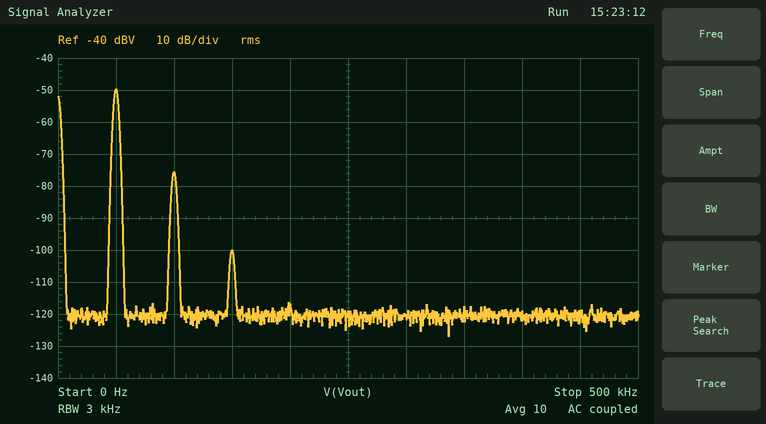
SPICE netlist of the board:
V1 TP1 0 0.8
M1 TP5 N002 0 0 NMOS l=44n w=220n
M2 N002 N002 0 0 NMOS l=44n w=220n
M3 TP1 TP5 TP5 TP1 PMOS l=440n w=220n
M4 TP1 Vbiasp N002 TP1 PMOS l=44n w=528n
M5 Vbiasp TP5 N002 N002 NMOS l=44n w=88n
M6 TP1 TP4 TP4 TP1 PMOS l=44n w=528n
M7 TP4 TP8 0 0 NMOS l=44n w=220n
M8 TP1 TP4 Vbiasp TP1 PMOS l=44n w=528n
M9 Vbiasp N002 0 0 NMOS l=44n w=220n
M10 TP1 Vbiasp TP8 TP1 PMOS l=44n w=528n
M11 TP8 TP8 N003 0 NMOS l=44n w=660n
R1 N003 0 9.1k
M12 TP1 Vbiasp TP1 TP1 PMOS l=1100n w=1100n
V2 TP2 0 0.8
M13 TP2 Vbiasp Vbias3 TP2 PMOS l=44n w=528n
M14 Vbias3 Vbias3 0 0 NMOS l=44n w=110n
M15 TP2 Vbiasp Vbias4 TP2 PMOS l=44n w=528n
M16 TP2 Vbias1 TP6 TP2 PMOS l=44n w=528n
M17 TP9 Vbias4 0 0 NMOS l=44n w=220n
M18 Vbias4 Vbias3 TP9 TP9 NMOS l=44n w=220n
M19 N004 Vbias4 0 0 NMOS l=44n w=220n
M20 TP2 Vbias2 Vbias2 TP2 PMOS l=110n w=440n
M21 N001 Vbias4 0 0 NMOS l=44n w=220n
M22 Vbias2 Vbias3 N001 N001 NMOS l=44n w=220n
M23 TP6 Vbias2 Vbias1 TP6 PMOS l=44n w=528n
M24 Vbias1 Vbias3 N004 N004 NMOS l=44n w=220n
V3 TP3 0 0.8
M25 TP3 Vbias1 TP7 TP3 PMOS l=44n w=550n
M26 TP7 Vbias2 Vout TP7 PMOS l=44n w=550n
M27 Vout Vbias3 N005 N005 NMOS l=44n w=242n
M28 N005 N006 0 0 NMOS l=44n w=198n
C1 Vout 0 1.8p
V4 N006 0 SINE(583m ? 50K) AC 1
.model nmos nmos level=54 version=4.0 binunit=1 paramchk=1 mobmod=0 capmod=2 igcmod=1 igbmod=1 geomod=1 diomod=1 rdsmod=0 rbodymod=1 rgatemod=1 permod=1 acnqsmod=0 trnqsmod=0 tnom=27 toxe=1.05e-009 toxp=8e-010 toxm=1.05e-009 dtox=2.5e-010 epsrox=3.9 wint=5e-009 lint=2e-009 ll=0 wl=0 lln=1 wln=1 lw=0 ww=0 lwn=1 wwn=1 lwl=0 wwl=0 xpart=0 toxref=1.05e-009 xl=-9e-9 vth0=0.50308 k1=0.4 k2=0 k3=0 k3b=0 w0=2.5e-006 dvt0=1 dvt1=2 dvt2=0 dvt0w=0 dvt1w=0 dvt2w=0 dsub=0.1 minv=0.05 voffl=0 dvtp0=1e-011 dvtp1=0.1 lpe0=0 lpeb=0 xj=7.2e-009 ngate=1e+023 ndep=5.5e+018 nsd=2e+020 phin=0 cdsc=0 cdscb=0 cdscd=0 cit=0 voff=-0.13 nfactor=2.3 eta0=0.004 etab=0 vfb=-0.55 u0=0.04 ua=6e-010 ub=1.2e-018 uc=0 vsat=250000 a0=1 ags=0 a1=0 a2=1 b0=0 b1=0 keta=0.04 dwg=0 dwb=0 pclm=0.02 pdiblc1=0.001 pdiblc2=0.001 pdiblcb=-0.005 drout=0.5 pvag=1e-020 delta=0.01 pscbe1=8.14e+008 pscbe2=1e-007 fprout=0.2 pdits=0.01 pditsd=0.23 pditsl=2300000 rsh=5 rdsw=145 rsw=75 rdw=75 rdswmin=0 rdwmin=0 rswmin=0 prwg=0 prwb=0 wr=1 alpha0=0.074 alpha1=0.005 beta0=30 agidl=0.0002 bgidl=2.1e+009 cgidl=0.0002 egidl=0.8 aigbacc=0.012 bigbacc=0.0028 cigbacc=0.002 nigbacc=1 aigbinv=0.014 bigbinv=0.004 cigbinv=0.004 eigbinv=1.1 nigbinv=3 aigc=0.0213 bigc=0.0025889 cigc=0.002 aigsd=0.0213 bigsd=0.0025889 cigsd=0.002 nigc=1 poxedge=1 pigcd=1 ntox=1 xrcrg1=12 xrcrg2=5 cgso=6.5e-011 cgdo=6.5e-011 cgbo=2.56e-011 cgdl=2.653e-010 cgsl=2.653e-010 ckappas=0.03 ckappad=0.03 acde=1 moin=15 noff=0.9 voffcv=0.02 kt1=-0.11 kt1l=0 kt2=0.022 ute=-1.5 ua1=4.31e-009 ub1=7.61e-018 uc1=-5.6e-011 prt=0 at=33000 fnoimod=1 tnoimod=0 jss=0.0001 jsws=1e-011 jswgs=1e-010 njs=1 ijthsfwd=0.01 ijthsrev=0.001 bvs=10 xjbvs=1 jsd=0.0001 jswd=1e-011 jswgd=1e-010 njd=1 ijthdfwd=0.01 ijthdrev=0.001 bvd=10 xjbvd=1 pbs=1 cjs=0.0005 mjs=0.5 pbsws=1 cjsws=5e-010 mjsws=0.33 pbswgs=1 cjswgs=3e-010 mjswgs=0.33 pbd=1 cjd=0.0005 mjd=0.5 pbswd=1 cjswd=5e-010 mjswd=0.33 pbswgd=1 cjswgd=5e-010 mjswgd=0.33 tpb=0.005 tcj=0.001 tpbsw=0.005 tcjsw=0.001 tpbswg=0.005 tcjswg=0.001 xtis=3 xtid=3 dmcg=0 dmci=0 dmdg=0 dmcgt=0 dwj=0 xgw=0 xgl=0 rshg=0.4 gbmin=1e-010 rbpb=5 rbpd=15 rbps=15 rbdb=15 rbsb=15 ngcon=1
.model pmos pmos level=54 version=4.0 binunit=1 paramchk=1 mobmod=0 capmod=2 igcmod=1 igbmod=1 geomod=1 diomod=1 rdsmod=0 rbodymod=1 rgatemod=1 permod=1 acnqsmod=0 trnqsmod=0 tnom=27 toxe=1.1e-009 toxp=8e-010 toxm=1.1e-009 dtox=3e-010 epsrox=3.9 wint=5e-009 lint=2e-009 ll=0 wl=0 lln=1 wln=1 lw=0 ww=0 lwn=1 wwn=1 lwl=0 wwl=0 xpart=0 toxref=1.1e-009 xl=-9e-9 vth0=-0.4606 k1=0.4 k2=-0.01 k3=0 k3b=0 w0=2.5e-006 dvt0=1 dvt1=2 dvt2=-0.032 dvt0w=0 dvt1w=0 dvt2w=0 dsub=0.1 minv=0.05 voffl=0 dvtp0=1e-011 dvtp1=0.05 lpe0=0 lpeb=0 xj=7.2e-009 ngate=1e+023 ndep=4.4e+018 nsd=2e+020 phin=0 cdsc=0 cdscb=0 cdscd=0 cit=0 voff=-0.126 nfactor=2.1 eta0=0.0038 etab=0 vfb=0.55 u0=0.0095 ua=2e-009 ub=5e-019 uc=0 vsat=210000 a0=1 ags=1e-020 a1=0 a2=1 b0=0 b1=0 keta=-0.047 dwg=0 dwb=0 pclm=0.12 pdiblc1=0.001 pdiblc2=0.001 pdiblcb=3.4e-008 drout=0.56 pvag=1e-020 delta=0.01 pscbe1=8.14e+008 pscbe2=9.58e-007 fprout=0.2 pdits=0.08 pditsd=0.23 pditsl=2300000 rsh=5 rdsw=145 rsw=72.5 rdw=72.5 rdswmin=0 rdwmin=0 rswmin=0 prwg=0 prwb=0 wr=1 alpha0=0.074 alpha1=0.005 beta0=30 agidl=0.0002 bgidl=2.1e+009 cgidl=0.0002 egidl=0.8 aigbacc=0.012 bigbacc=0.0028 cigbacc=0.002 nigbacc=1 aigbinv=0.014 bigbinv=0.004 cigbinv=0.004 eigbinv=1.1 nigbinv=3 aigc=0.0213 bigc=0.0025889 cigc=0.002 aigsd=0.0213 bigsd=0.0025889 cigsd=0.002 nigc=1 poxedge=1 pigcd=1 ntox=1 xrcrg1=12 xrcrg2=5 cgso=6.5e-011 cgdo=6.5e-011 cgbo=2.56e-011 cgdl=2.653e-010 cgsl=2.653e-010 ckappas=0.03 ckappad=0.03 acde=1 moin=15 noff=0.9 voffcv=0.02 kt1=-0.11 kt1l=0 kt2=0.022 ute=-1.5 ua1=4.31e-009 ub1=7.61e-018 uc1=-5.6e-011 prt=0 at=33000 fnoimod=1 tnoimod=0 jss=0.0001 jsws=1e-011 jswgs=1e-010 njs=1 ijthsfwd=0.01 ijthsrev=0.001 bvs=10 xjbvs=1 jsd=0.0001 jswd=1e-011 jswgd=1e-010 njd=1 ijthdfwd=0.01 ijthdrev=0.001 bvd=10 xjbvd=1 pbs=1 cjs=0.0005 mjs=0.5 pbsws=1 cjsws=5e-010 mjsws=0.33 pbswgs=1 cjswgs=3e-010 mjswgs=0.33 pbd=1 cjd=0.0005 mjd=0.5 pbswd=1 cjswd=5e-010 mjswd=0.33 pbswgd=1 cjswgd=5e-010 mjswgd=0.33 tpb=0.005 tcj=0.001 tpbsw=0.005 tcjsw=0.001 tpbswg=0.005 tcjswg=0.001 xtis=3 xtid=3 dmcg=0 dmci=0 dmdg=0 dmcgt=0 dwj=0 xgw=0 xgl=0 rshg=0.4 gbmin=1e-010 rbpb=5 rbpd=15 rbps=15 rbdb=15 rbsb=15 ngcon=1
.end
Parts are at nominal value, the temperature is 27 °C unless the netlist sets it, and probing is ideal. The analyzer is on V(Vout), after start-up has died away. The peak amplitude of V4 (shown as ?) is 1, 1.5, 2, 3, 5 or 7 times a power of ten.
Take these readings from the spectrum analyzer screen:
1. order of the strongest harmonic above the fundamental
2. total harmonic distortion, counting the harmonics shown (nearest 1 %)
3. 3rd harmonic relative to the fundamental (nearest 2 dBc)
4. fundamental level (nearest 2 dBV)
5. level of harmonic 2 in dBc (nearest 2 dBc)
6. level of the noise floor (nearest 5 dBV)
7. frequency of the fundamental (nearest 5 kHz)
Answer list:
2
5 %
-50 dBc
-50 dBV
-26 dBc
-120 dBV
50 kHz
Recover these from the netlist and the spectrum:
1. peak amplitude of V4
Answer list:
5 mV
